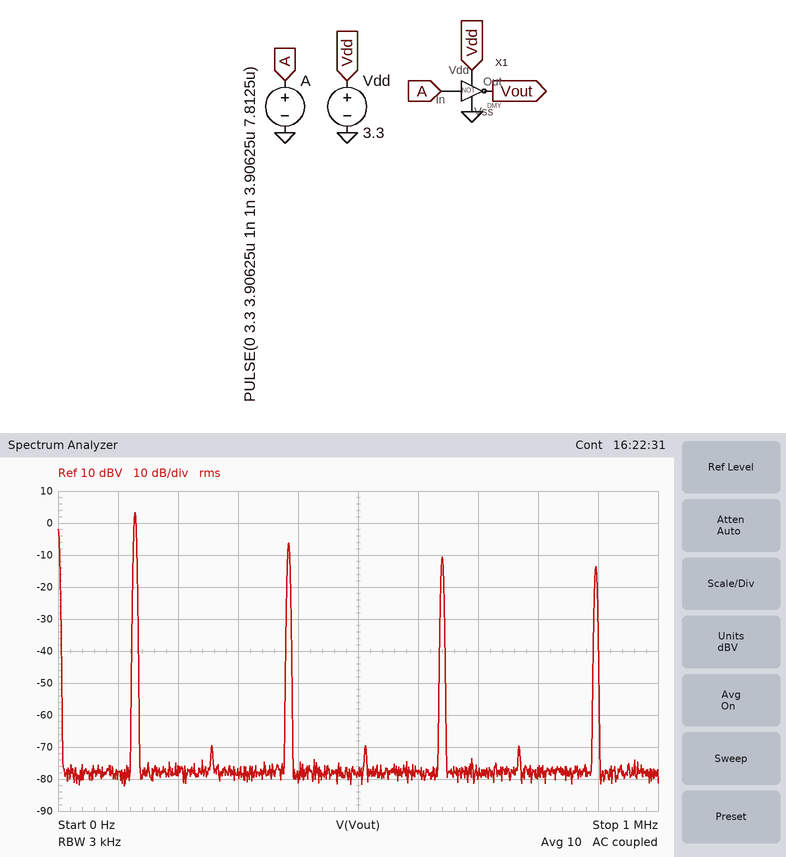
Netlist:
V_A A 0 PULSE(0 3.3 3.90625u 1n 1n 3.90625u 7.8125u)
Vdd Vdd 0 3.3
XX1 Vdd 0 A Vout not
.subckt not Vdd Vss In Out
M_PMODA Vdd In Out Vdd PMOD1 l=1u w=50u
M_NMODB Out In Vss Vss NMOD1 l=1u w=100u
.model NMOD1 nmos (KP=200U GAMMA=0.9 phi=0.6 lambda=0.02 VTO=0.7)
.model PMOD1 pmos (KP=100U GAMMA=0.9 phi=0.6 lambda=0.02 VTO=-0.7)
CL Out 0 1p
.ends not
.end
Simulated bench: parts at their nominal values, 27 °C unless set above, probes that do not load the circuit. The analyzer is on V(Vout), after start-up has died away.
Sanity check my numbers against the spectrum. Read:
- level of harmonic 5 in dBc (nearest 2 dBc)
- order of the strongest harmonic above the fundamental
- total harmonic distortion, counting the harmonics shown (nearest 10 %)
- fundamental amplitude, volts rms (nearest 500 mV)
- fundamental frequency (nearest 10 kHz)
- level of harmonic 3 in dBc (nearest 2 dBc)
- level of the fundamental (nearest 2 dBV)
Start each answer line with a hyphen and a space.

- -14 dBc
- 3
- 40 %
- 1.5 V
- 130 kHz
- -10 dBc
- 4 dBV
